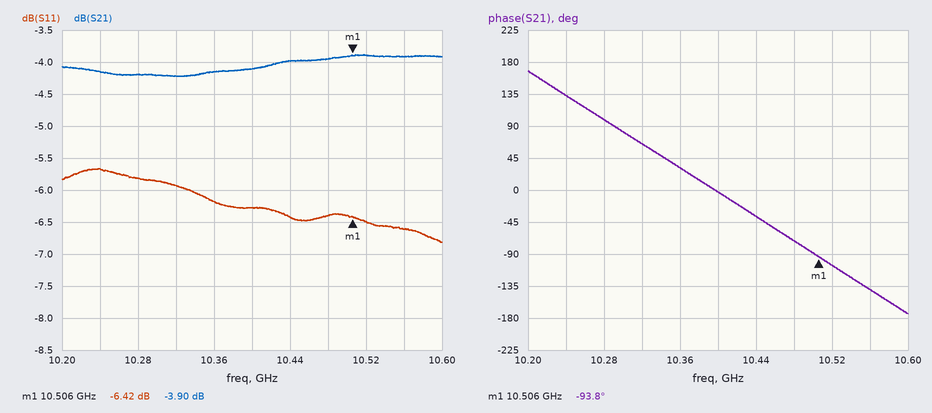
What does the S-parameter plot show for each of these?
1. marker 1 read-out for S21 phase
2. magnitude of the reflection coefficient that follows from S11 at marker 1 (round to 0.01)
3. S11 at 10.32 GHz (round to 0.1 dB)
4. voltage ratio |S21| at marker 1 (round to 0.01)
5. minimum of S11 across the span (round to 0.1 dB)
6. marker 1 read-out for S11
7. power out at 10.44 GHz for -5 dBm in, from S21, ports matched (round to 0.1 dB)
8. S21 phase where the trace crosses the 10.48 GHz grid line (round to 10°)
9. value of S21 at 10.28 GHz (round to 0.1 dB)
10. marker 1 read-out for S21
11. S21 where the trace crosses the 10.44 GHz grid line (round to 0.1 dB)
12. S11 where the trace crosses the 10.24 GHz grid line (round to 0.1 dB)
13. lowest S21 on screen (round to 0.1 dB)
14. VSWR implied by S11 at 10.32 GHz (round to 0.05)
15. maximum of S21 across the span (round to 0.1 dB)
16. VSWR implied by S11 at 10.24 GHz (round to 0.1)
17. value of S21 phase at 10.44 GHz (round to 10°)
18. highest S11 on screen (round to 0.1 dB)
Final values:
-93.8°
0.48
-5.9 dB
0.64
-6.8 dB
-6.42 dB
-9.0 dBm
-70°
-4.2 dB
-3.90 dB
-4.0 dB
-5.7 dB
-4.2 dB
3.05
-3.9 dB
3.2
-40°
-5.7 dB
